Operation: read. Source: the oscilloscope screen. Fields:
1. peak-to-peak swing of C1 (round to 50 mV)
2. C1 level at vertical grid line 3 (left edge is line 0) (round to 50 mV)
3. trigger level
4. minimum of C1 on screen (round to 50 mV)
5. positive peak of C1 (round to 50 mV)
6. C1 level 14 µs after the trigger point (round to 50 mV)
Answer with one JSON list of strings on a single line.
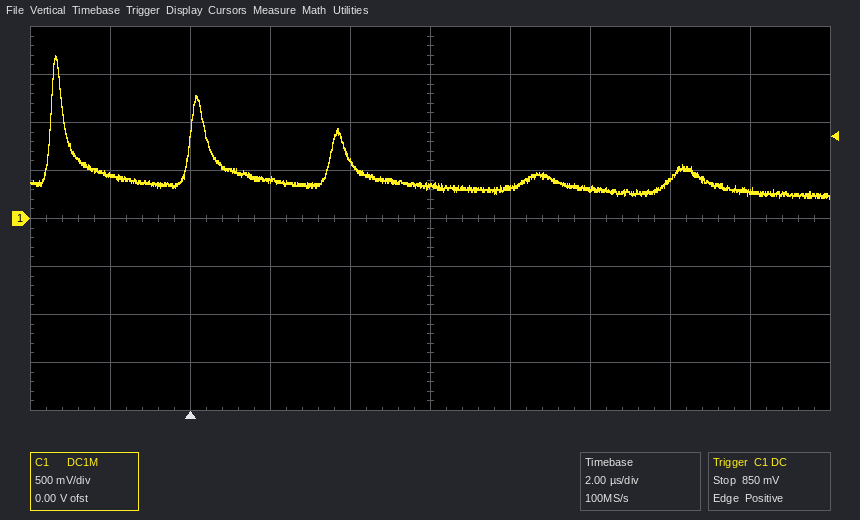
["1.50 V", "400 mV", "850 mV", "200 mV", "1.70 V", "300 mV"]
